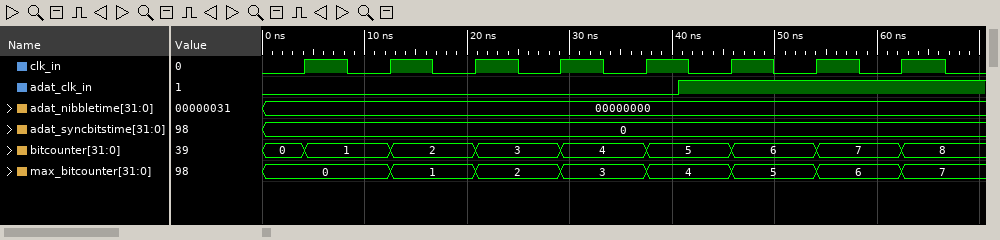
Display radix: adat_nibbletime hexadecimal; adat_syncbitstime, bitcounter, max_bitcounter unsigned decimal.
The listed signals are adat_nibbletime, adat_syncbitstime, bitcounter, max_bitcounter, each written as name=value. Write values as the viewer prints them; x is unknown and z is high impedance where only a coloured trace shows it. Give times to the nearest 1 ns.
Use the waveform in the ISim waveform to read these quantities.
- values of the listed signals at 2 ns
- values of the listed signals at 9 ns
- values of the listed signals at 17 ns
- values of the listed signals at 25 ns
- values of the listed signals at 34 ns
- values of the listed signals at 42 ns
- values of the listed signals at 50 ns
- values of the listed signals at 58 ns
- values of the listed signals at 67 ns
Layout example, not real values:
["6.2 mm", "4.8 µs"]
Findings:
["adat_nibbletime=00000000, adat_syncbitstime=0, bitcounter=0, max_bitcounter=0", "adat_nibbletime=00000000, adat_syncbitstime=0, bitcounter=1, max_bitcounter=0", "adat_nibbletime=00000000, adat_syncbitstime=0, bitcounter=2, max_bitcounter=1", "adat_nibbletime=00000000, adat_syncbitstime=0, bitcounter=3, max_bitcounter=2", "adat_nibbletime=00000000, adat_syncbitstime=0, bitcounter=4, max_bitcounter=3", "adat_nibbletime=00000000, adat_syncbitstime=0, bitcounter=5, max_bitcounter=4", "adat_nibbletime=00000000, adat_syncbitstime=0, bitcounter=6, max_bitcounter=5", "adat_nibbletime=00000000, adat_syncbitstime=0, bitcounter=7, max_bitcounter=6", "adat_nibbletime=00000000, adat_syncbitstime=0, bitcounter=8, max_bitcounter=7"]
